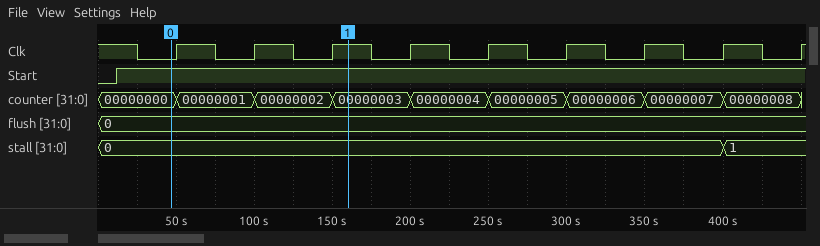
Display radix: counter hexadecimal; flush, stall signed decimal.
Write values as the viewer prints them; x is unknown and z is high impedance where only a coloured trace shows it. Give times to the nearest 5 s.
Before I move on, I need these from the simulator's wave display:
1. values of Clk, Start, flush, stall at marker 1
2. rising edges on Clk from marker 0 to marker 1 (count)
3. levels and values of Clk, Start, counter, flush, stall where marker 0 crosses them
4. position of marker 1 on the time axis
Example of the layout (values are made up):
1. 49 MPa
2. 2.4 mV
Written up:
1. Clk=1, Start=1, flush=0, stall=0
2. 3
3. Clk=0, Start=1, counter=00000000, flush=0, stall=0
4. 160 s
